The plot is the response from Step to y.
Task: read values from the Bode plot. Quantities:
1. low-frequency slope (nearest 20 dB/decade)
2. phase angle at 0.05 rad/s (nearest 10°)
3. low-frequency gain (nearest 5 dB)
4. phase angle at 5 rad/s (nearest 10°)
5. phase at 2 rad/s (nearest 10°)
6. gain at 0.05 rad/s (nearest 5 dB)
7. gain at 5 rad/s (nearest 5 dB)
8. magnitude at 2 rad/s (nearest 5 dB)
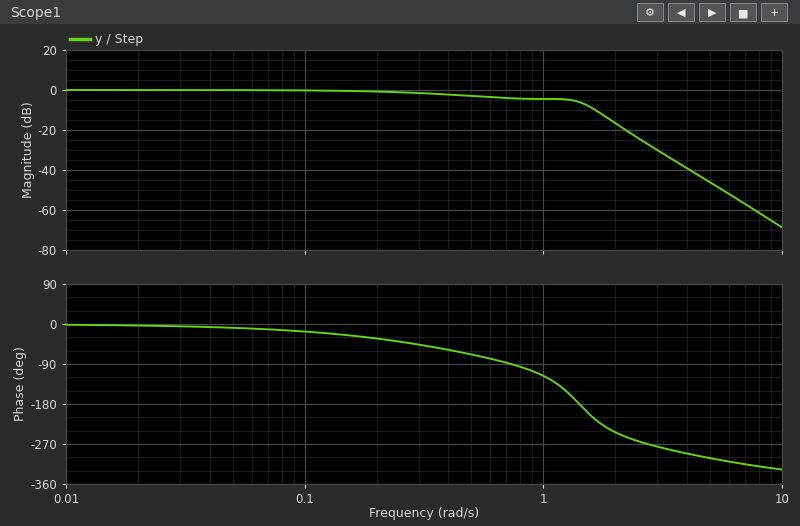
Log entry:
0 dB/decade
-10°
0 dB
-300°
-240°
0 dB
-45 dB
-15 dB
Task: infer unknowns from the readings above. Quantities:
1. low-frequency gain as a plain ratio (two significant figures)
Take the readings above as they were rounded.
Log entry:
1.0
